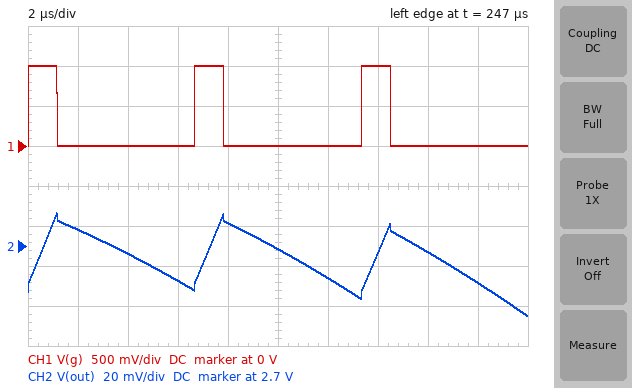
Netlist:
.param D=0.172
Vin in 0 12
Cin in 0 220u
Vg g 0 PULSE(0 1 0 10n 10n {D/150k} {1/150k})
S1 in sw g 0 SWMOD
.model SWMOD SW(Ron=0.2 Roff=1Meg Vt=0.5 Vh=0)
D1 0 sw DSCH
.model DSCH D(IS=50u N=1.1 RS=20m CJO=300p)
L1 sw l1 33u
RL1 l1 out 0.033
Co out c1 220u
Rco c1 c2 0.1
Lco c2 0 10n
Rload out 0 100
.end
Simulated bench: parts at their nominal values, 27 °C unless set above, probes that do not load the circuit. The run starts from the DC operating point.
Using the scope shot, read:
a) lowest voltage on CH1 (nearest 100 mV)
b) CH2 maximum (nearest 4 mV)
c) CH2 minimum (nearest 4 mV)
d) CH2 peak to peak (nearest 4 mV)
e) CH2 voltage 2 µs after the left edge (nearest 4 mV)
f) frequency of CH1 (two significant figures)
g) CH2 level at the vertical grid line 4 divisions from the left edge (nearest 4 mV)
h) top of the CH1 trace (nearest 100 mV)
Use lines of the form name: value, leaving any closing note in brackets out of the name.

lowest voltage on CH1: 0 V
CH2 maximum: 2.716 V
CH2 minimum: 2.664 V
CH2 peak to peak: 52 mV
CH2 voltage 2 µs after the left edge: 2.708 V
frequency of CH1: 150 kHz
CH2 level at the vertical grid line 4 divisions from the left edge: 2.712 V
top of the CH1 trace: 1.0 V
